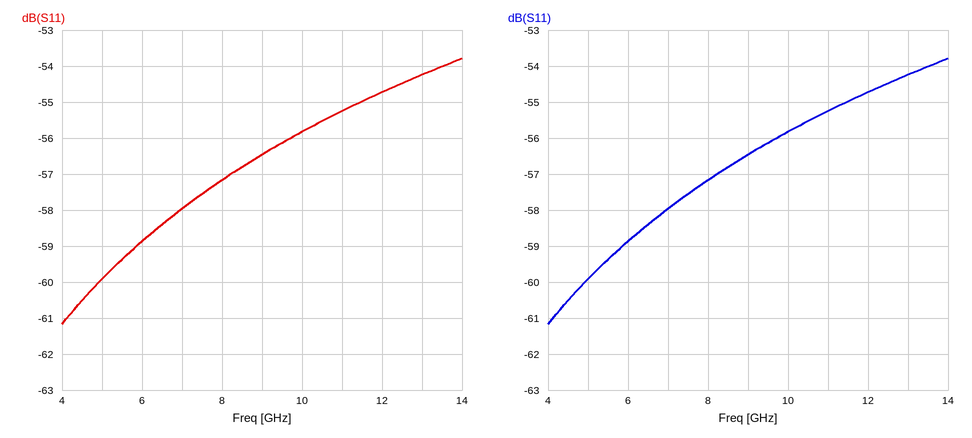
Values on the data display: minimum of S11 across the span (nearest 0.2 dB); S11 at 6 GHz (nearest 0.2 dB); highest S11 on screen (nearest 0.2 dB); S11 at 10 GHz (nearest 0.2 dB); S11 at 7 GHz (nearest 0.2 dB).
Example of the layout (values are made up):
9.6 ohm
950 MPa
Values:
-61.2 dB
-58.8 dB
-53.8 dB
-55.8 dB
-58.0 dB
